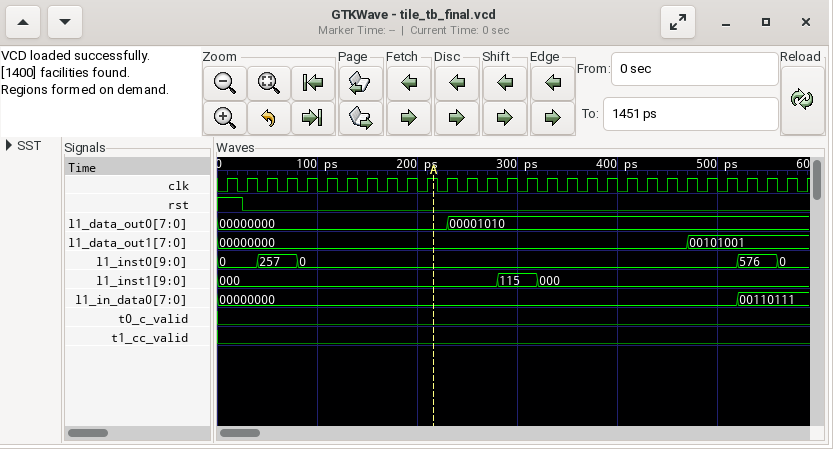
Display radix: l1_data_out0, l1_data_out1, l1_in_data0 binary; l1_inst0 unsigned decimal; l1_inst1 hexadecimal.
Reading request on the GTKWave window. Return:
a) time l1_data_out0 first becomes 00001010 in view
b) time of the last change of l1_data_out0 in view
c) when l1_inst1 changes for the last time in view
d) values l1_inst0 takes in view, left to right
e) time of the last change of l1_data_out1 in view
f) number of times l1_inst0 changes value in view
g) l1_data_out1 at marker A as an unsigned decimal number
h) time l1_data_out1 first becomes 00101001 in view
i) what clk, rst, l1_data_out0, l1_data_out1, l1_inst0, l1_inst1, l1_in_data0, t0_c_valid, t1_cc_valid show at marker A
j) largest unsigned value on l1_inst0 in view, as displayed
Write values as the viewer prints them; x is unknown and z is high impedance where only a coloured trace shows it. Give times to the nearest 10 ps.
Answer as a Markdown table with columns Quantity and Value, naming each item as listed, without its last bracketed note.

| Quantity | Value |
|---|---|
| time l1_data_out0 first becomes 00001010 in view | 230 ps |
| time of the last change of l1_data_out0 in view | 230 ps |
| when l1_inst1 changes for the last time in view | 320 ps |
| values l1_inst0 takes in view, left to right | 0, 257, 0, 576, 0 |
| time of the last change of l1_data_out1 in view | 470 ps |
| number of times l1_inst0 changes value in view | 4 |
| l1_data_out1 at marker A as an unsigned decimal number | 0 |
| time l1_data_out1 first becomes 00101001 in view | 470 ps |
| what clk, rst, l1_data_out0, l1_data_out1, l1_inst0, l1_inst1, l1_in_data0, t0_c_valid, t1_cc_valid show at marker A | clk=1, rst=0, l1_data_out0=00000000, l1_data_out1=00000000, l1_inst0=0, l1_inst1=000, l1_in_data0=00000000, t0_c_valid=0, t1_cc_valid=0 |
| largest unsigned value on l1_inst0 in view, as displayed | 576 |
